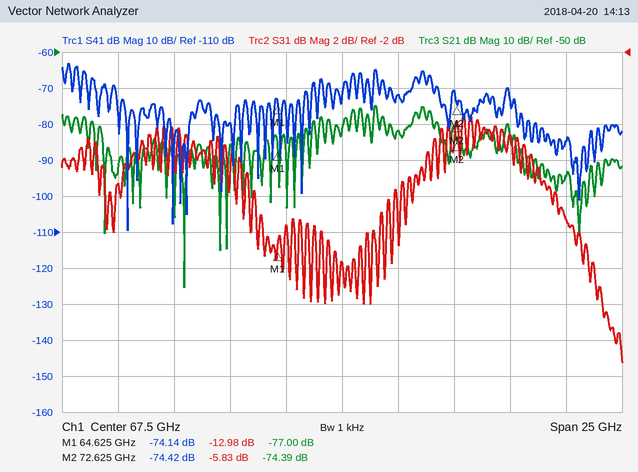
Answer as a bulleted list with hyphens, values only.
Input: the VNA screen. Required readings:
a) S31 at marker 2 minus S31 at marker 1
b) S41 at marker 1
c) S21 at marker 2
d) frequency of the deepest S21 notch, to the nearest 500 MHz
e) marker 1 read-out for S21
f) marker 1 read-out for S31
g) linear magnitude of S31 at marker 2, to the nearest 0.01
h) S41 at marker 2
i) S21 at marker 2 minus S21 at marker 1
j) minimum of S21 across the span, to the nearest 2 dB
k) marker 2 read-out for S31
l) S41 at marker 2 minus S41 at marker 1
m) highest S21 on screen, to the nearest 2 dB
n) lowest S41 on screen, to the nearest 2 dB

- 7.15 dB
- -74.14 dB
- -74.39 dB
- 60.5 GHz
- -77.00 dB
- -12.98 dB
- 0.51
- -74.42 dB
- 2.61 dB
- -116 dB
- -5.83 dB
- -0.28 dB
- -64 dB
- -110 dB
